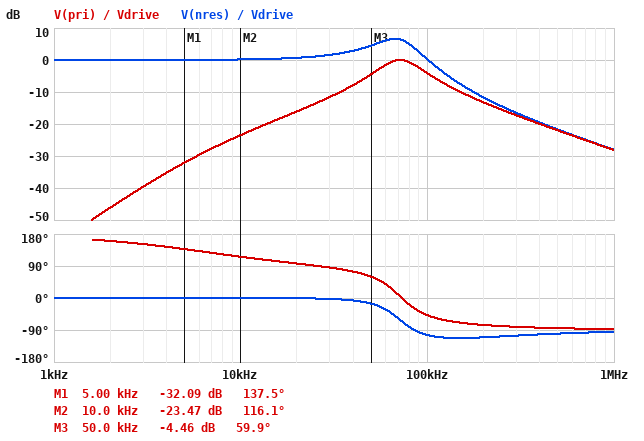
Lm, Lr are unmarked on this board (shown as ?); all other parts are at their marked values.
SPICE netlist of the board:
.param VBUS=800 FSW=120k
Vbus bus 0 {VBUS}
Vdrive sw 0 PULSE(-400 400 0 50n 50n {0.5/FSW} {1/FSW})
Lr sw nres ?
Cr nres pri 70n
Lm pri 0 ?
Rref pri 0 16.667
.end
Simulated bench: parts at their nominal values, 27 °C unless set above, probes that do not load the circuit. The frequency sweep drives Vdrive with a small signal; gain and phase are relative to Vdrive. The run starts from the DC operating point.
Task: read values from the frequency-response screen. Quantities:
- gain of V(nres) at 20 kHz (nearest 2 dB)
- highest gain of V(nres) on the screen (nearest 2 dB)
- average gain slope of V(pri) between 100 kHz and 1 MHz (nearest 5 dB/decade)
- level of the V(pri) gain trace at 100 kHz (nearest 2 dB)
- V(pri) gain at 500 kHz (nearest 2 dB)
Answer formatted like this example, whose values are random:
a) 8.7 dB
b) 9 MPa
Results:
a) 0 dB
b) 6 dB
c) -25 dB/decade
d) -4 dB
e) -22 dB
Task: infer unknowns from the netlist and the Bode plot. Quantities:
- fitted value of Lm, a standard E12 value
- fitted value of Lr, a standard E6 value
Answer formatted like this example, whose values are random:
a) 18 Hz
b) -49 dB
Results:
a) 470 µH
b) 68 µH
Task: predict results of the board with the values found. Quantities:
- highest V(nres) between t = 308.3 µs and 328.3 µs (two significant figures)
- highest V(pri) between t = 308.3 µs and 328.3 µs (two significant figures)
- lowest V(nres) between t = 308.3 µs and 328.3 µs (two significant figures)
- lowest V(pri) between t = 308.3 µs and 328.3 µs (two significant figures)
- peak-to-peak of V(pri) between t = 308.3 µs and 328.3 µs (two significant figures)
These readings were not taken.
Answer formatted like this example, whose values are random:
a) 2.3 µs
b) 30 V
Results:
a) 360 V
b) 240 V
c) -350 V
d) -240 V
e) 480 V
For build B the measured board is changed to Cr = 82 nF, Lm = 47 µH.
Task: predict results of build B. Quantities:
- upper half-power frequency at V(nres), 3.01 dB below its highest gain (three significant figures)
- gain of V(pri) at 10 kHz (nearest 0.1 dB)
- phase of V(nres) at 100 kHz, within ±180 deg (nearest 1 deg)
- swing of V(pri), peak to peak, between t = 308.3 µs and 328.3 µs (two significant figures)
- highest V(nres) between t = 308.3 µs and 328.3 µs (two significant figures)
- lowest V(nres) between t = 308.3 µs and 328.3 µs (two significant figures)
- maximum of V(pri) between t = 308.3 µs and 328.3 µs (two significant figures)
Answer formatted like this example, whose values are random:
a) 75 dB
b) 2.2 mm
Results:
a) 63.7 kHz
b) -36.2 dB
c) -112 deg
d) 340 V
e) 230 V
f) -220 V
g) 170 V
